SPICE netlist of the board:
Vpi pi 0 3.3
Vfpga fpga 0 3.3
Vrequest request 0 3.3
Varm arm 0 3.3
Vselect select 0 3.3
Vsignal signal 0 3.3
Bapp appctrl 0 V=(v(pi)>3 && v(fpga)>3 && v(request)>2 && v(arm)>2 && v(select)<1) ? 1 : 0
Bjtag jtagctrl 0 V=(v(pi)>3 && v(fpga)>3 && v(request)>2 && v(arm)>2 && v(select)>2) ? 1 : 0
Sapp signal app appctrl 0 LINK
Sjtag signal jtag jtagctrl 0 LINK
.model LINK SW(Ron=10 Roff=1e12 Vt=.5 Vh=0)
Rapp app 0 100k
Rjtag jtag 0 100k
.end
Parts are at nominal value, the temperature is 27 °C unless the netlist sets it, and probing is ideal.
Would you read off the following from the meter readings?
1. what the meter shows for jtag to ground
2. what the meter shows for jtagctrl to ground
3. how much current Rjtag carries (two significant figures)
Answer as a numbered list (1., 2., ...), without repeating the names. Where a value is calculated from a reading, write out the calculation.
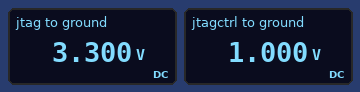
1. 3.300 V
2. 1.000 V
3. (3.3 V) / 100 kΩ = 33 µA
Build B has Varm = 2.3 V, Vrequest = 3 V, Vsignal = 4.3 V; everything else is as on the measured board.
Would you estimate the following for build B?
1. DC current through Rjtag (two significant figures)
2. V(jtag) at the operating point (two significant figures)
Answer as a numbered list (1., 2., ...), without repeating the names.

1. 43 µA
2. 4.3 V
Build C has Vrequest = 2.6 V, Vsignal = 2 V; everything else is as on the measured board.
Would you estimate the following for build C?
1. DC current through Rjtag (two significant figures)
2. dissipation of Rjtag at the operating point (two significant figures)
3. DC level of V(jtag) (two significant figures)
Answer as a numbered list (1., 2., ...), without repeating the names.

1. 20 µA
2. 40 µW
3. 2.0 V
